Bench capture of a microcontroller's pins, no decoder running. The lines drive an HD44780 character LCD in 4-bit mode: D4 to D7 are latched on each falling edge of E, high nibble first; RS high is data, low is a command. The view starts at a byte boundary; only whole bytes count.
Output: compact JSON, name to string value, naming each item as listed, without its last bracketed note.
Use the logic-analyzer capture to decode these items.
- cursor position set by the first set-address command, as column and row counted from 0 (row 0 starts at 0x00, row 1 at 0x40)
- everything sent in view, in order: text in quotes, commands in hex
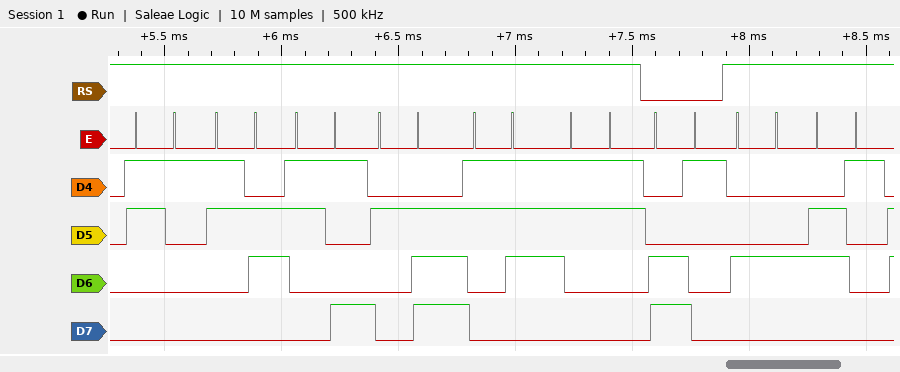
{"cursor position set by the first set-address command, as column and row counted from 0": "column 1, row 1", "everything sent in view, in order: text in quotes, commands in hex": "\"169.73\" 0xC1 \"Da\""}
